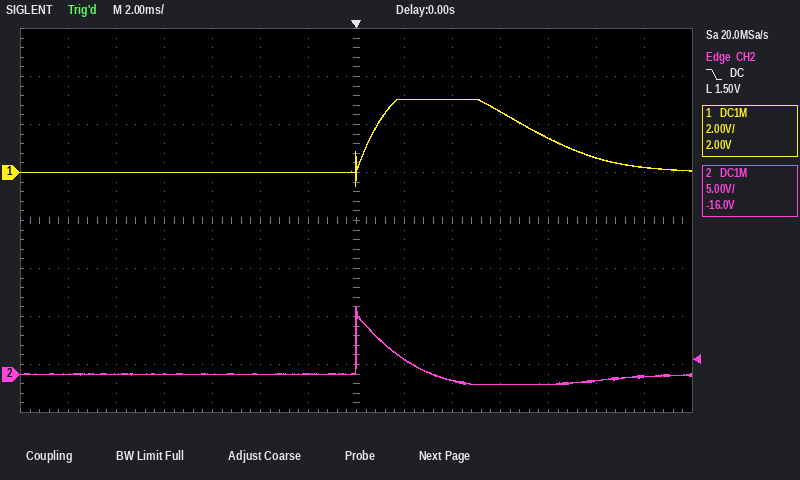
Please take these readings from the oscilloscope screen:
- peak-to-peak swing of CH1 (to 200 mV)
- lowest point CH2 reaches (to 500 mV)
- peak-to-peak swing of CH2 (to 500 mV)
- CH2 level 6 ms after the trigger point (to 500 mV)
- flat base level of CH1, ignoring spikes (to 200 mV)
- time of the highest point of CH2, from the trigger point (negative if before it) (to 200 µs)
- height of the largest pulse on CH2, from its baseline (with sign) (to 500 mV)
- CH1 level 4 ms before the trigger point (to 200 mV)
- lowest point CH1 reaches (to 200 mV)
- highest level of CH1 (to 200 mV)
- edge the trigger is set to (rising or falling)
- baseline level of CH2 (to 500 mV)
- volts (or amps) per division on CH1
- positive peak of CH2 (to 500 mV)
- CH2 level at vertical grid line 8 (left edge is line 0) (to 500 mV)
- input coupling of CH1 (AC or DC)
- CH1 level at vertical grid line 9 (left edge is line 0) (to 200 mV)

3.6 V
-1.0 V
8.0 V
-1.0 V
0.0 V
0.0 ms
+7.0 V
0.0 V
-600 mV
3.0 V
falling
0.0 V
2 V
7.0 V
1.5 V
DC
3.0 V
